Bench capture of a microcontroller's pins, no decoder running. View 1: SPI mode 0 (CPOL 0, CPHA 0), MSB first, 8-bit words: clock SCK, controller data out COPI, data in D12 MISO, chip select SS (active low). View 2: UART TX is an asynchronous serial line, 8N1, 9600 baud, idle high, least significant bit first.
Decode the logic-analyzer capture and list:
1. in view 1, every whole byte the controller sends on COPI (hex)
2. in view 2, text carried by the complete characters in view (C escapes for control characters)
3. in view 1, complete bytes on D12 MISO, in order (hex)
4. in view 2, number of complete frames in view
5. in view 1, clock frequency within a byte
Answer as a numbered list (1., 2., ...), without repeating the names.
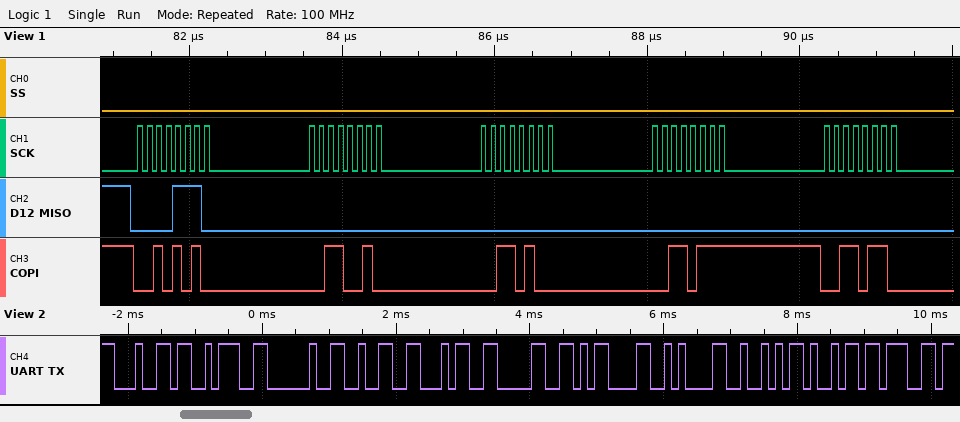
1. 2A 32 34 37 36
2. "d: 240\r\nRig"
3. 0E 00 00 00 00
4. 11
5. 8 MHz
